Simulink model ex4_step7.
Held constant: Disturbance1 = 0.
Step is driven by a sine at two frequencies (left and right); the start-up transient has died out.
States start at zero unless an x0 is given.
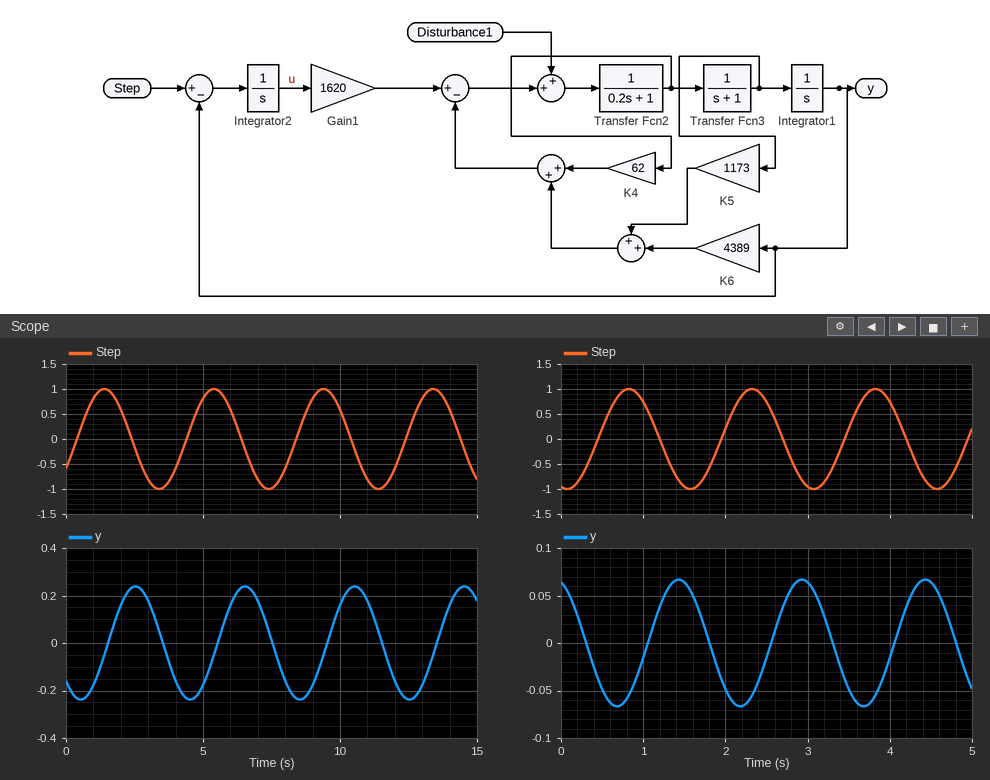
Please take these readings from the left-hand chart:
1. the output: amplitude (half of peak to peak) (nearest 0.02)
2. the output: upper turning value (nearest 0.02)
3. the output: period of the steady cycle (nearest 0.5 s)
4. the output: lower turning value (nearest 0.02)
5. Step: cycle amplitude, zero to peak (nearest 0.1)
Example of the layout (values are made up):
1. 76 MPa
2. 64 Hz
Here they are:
1. 0.24
2. 0.24
3. 4.0 s
4. -0.24
5. 1.0
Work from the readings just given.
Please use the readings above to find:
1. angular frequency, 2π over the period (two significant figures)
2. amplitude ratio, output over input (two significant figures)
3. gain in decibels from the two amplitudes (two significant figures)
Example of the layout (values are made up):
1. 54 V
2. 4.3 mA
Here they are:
1. 1.6 rad/s
2. 0.24
3. -12 dB
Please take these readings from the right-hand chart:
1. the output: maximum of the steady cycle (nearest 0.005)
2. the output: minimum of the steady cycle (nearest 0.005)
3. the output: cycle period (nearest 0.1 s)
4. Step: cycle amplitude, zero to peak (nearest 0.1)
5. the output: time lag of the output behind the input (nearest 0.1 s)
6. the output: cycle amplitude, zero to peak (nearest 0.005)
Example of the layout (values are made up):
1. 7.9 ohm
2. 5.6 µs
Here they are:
1. 0.065
2. -0.065
3. 1.5 s
4. 1.0
5. 0.6 s
6. 0.065
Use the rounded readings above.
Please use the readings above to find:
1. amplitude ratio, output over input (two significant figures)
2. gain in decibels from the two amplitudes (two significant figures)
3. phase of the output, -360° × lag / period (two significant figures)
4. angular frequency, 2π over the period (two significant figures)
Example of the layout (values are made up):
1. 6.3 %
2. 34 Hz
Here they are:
1. 0.065
2. -24 dB
3. -140°
4. 4.2 rad/s
